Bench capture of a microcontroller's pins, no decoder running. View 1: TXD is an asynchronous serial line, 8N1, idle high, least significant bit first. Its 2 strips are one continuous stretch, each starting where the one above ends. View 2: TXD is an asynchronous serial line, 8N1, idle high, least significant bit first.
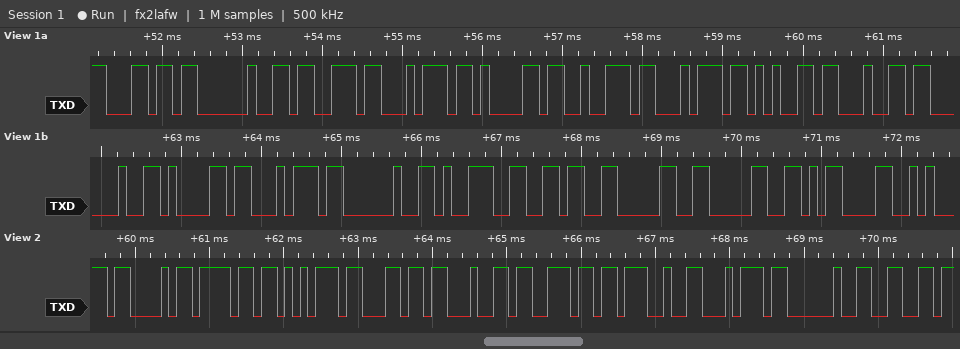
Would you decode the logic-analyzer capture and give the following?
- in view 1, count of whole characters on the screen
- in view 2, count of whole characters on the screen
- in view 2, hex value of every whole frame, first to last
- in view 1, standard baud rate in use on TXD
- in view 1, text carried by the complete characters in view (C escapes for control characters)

18
10
43 6F 75 6C 64 6E 27 74 20 66
9600 baud
"l started at 9600\r"
